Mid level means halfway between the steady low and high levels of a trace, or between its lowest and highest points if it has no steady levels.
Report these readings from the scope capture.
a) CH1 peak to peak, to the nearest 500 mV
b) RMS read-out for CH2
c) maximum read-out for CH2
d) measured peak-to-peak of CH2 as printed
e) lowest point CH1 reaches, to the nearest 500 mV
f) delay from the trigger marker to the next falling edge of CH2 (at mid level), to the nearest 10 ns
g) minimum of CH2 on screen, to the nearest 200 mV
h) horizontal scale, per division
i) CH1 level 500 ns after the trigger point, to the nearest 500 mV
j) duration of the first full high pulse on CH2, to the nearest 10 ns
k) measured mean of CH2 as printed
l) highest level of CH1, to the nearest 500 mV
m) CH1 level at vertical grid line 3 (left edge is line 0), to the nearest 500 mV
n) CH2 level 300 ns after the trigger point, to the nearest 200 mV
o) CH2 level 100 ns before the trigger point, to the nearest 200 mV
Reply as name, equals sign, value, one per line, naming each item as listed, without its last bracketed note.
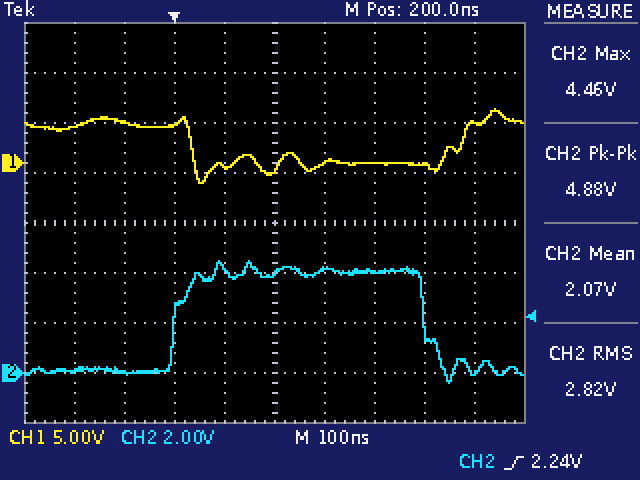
CH1 peak to peak, to the nearest 500 mV = 7.5 V
RMS read-out for CH2 = 2.82 V
maximum read-out for CH2 = 4.46 V
measured peak-to-peak of CH2 as printed = 4.88 V
lowest point CH1 reaches, to the nearest 500 mV = -2.0 V
delay from the trigger marker to the next falling edge of CH2 (at mid level), to the nearest 10 ns = 500 ns
minimum of CH2 on screen, to the nearest 200 mV = -400 mV
horizontal scale, per division = 100 ns
CH1 level 500 ns after the trigger point, to the nearest 500 mV = 0.0 V
duration of the first full high pulse on CH2, to the nearest 10 ns = 500 ns
measured mean of CH2 as printed = 2.07 V
highest level of CH1, to the nearest 500 mV = 5.5 V
CH1 level at vertical grid line 3 (left edge is line 0), to the nearest 500 mV = 4.0 V
CH2 level 300 ns after the trigger point, to the nearest 200 mV = 4.2 V
CH2 level 100 ns before the trigger point, to the nearest 200 mV = 0.0 V
